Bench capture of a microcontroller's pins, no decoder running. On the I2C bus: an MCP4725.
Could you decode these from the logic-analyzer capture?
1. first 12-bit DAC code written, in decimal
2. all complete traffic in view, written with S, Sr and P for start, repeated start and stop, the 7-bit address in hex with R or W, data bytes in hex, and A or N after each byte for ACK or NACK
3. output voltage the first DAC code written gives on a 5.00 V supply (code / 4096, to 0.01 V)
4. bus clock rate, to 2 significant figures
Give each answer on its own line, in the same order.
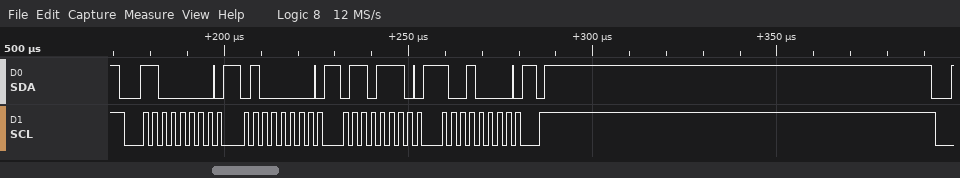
1769
S 60W A 40 A 6E A 90 A P
2.16 V
400 kHz
